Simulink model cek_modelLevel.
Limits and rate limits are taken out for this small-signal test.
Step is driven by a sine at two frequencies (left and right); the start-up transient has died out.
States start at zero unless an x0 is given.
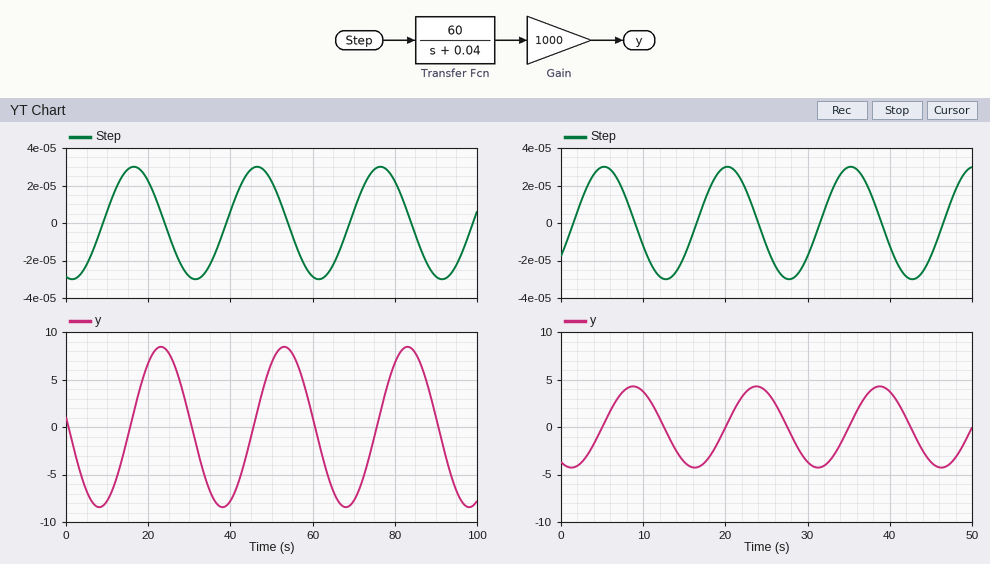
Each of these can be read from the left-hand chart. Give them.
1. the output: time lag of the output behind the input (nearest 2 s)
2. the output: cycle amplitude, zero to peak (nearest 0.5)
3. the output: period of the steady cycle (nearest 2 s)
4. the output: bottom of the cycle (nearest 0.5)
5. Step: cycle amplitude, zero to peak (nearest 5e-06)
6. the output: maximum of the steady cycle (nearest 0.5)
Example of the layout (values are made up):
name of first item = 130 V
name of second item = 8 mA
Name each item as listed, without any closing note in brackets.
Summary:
the output: time lag of the output behind the input = 6 s
the output: cycle amplitude, zero to peak = 8.5
the output: period of the steady cycle = 30 s
the output: bottom of the cycle = -8.5
Step: cycle amplitude, zero to peak = 0.000030
the output: maximum of the steady cycle = 8.5
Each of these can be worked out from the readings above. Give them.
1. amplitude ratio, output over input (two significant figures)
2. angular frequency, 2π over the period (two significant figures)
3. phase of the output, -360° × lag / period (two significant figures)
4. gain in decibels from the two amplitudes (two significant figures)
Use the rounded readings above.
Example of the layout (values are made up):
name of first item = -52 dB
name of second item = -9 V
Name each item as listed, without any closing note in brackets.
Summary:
amplitude ratio, output over input = 280000
angular frequency, 2π over the period = 0.21 rad/s
phase of the output, -360° × lag / period = -72°
gain in decibels from the two amplitudes = 110 dB
